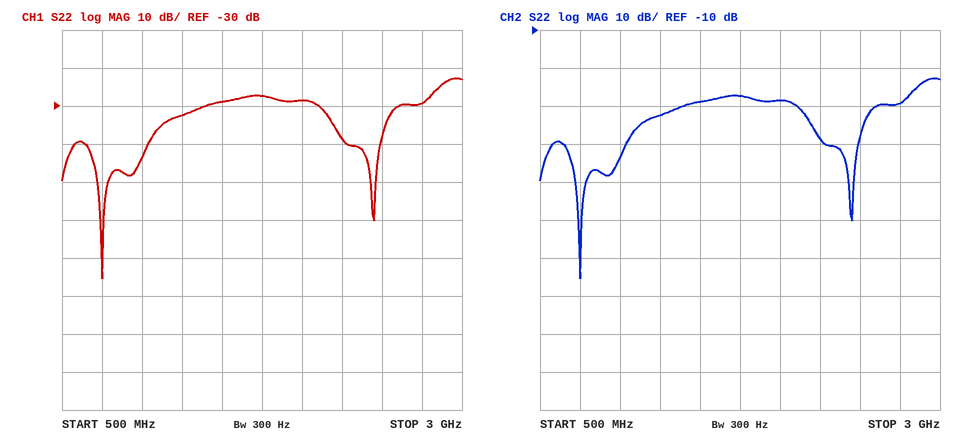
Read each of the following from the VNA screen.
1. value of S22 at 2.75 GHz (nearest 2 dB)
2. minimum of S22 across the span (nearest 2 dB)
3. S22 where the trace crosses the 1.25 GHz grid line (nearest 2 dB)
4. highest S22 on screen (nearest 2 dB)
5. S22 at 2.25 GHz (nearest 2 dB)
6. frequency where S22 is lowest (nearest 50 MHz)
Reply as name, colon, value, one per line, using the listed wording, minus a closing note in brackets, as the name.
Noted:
value of S22 at 2.75 GHz: -30 dB
minimum of S22 across the span: -76 dB
S22 where the trace crosses the 1.25 GHz grid line: -32 dB
highest S22 on screen: -22 dB
S22 at 2.25 GHz: -38 dB
frequency where S22 is lowest: 750 MHz
